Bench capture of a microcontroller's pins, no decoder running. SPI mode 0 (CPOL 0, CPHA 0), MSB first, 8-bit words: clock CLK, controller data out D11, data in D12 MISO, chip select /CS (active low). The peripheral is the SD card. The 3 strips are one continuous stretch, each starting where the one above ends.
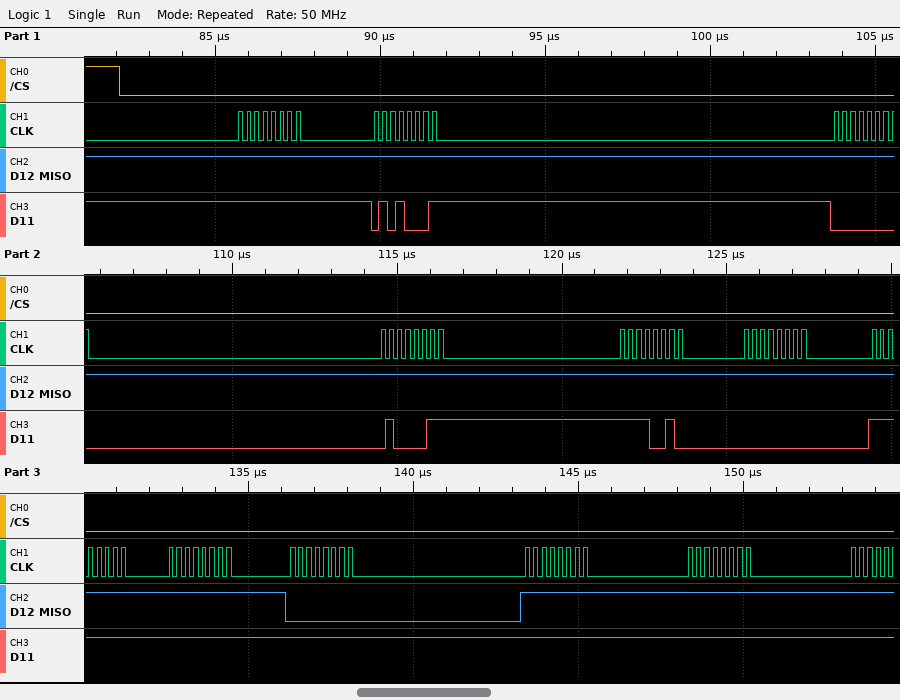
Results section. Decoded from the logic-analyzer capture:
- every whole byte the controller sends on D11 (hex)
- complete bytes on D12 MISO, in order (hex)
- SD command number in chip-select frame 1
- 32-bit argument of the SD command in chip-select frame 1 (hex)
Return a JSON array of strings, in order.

["0xFF 0x51 0x00 0x43 0xF2 0x00 0xFF 0xFF 0xFF 0xFF 0xFF", "0xFF 0xFF 0xFF 0xFF 0xFF 0xFF 0xFF 0xFF 0x00 0xFF 0xFF", "CMD17", "0x0043F200"]
